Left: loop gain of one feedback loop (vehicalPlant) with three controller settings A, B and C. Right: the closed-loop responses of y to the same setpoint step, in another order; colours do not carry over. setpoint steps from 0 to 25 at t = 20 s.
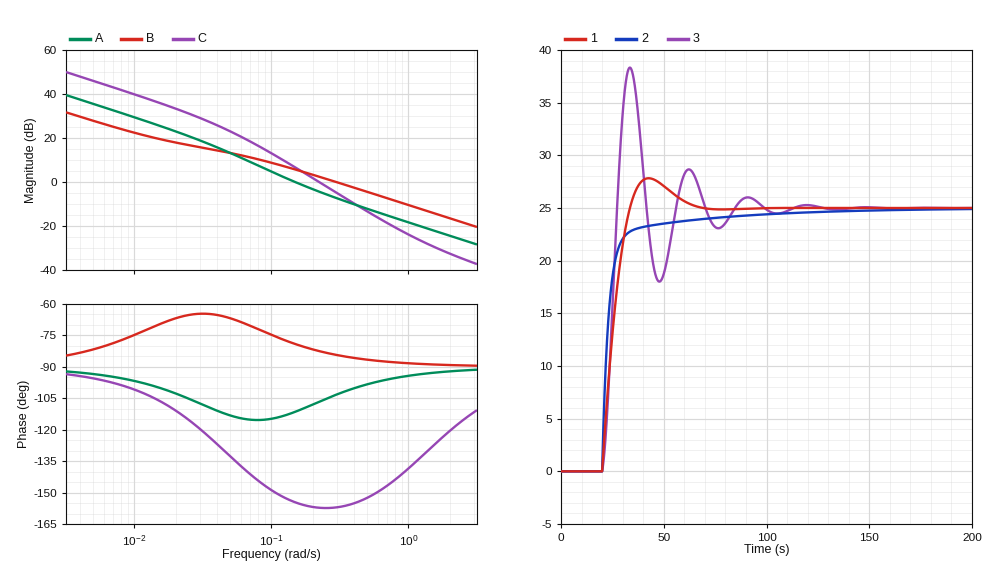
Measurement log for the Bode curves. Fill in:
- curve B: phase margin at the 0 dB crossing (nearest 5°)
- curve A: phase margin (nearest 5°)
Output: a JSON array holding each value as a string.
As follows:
["95°", "70°"]
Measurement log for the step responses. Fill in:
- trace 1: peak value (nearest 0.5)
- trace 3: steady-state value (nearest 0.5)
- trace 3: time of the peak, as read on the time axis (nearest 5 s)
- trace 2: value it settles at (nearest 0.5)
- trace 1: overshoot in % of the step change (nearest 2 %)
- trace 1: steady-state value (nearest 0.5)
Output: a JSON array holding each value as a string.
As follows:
["28.0", "25.0", "35 s", "25.0", "12 %", "25.0"]
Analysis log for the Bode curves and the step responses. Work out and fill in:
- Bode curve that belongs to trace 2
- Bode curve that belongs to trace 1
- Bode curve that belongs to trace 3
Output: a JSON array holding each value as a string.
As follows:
["B", "A", "C"]
